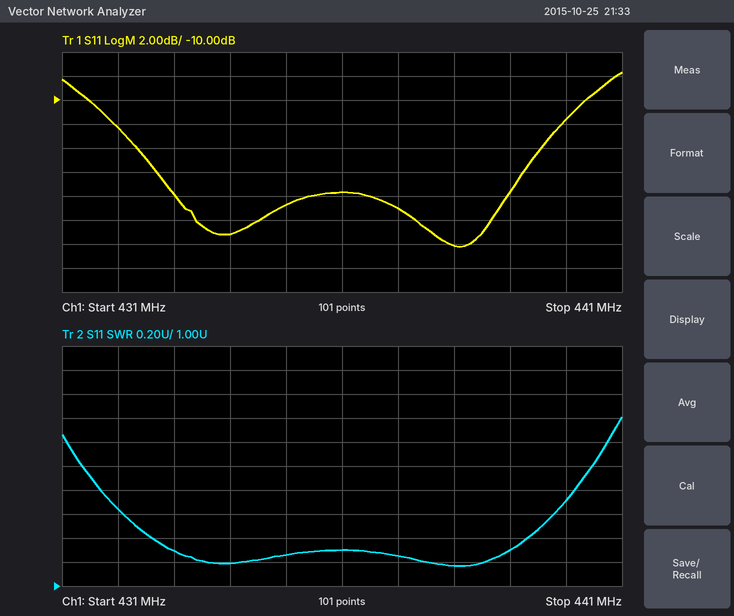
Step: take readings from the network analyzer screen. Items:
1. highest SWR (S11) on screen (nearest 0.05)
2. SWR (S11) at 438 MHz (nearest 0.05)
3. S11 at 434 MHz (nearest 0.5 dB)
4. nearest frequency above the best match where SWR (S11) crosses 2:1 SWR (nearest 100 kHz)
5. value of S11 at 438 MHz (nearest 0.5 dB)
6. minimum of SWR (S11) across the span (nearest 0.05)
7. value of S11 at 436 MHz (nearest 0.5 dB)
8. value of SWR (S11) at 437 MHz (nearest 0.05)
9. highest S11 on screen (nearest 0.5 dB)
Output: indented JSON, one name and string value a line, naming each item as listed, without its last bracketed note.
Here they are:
{
  "highest SWR (S11) on screen": "2.40",
  "SWR (S11) at 438 MHz": "1.15",
  "S11 at 434 MHz": "-21.0 dB",
  "nearest frequency above the best match where SWR (S11) crosses 2:1 SWR": "440.5 MHz",
  "value of S11 at 438 MHz": "-22.0 dB",
  "minimum of SWR (S11) across the span": "1.15",
  "value of S11 at 436 MHz": "-17.5 dB",
  "value of SWR (S11) at 437 MHz": "1.25",
  "highest S11 on screen": "-7.5 dB"
}
